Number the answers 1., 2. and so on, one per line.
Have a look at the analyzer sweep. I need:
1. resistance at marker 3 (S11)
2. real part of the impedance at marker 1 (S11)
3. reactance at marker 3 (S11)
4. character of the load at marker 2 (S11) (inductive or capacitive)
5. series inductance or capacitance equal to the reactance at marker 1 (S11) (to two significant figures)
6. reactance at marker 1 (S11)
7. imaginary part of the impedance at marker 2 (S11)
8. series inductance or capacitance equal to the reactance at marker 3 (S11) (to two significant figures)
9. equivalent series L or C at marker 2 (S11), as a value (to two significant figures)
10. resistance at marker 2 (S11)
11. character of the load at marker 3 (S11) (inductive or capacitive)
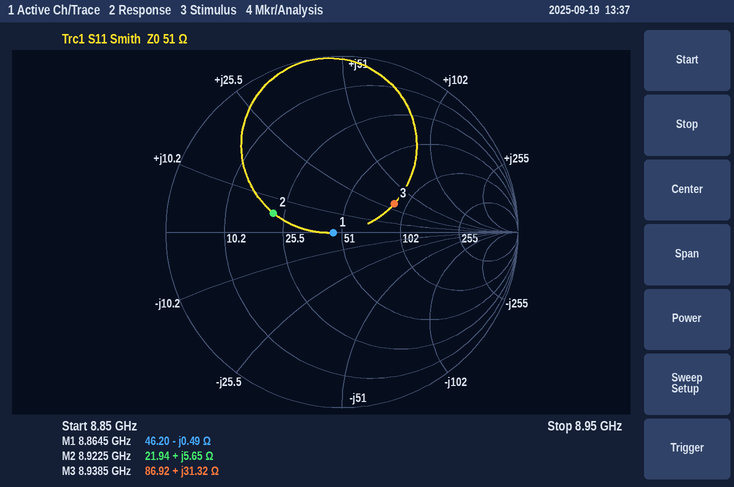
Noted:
1. 86.92 Ω
2. 46.20 Ω
3. +31.32 Ω
4. inductive
5. 37 pF
6. -0.49 Ω
7. +5.65 Ω
8. 560 pH
9. 100 pH
10. 21.94 Ω
11. inductive
